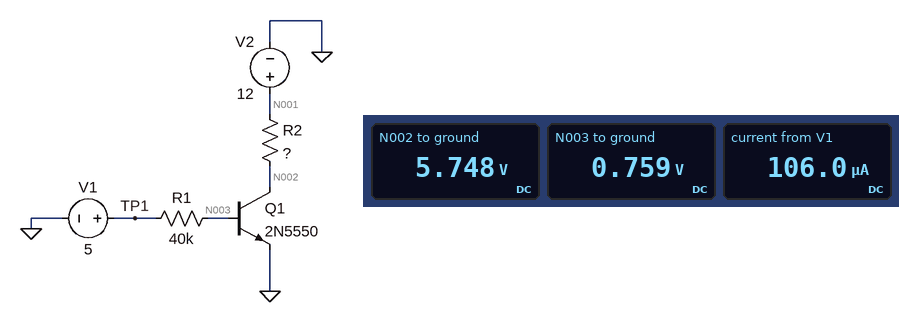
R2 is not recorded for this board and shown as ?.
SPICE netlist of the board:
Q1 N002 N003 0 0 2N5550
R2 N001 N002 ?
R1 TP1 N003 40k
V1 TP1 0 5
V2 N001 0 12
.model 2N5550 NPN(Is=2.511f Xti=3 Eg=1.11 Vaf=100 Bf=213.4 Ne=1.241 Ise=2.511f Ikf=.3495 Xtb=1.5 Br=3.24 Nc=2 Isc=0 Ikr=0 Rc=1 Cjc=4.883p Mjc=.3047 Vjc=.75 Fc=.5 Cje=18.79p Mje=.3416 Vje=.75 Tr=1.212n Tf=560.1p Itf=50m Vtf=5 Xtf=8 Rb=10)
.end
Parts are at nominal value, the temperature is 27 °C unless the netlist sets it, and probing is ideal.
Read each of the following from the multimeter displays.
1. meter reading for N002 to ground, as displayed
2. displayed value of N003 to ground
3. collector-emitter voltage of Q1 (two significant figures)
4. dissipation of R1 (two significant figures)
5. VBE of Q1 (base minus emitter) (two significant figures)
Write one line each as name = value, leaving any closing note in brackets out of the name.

meter reading for N002 to ground, as displayed = 5.748 V
displayed value of N003 to ground = 0.759 V
collector-emitter voltage of Q1 = 5.7 V
dissipation of R1 = 450 µW
VBE of Q1 (base minus emitter) = 760 mV
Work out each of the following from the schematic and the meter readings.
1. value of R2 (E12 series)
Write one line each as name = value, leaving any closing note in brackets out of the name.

value of R2 = 470 Ω
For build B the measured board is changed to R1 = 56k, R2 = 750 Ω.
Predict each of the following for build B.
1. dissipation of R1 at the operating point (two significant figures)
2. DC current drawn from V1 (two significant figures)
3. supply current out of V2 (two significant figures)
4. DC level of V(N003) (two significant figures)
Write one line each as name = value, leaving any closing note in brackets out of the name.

dissipation of R1 at the operating point = 320 µW
DC current drawn from V1 = 76 µA
supply current out of V2 = 9.3 mA
DC level of V(N003) = 750 mV
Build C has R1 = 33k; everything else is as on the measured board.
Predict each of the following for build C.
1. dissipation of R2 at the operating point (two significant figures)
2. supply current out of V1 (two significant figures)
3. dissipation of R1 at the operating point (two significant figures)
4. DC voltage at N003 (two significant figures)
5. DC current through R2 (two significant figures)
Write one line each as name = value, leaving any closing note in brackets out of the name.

dissipation of R2 at the operating point = 120 mW
supply current out of V1 = 130 µA
dissipation of R1 at the operating point = 540 µW
DC voltage at N003 = 760 mV
DC current through R2 = 16 mA
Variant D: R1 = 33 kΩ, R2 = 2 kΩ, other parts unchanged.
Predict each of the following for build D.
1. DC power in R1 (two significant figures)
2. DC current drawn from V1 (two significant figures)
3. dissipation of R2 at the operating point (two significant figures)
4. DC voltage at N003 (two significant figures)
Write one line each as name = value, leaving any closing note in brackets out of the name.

DC power in R1 = 550 µW
DC current drawn from V1 = 130 µA
dissipation of R2 at the operating point = 71 mW
DC voltage at N003 = 740 mV
